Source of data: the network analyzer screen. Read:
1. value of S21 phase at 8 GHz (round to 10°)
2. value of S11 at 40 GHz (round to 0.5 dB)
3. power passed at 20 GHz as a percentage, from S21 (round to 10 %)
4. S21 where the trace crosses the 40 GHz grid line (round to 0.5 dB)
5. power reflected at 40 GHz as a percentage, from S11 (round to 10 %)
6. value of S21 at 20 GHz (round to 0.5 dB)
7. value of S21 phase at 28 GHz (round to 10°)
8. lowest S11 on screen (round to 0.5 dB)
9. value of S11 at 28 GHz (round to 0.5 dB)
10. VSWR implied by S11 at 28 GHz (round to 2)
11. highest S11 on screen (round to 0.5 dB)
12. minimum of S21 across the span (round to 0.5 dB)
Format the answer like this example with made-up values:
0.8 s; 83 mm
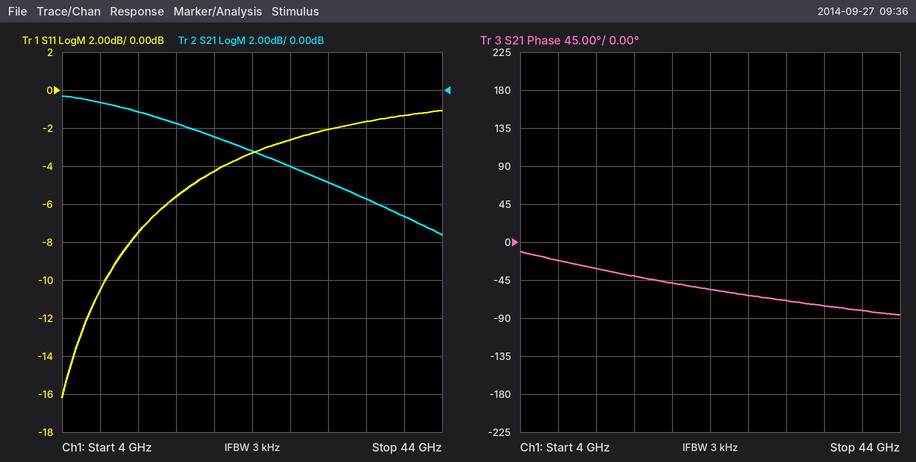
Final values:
-20°; -1.5 dB; 60 %; -6.5 dB; 70 %; -2.5 dB; -60°; -16.0 dB; -2.5 dB; 6; -1.0 dB; -7.5 dB
